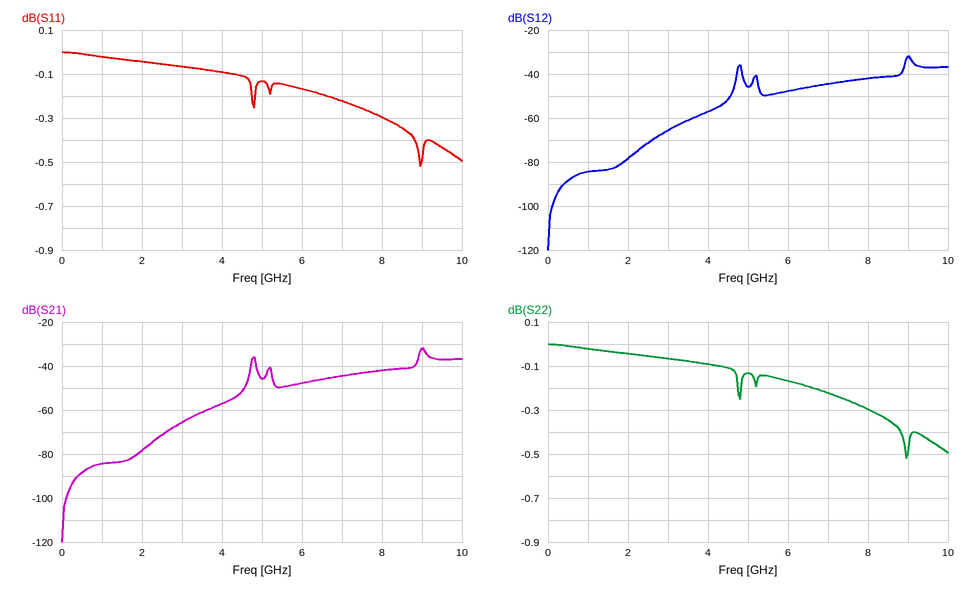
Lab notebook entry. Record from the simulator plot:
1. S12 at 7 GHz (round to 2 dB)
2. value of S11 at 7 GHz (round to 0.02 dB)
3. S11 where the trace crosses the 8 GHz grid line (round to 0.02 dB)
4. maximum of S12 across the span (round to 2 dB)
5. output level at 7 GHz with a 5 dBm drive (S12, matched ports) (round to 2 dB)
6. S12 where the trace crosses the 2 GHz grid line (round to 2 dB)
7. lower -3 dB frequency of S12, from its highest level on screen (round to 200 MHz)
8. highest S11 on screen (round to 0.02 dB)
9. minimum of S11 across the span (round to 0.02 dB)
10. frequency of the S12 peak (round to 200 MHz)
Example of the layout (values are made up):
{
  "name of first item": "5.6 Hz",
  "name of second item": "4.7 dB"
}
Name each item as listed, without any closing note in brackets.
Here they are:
{
  "S12 at 7 GHz": "-44 dB",
  "value of S11 at 7 GHz": "-0.22 dB",
  "S11 where the trace crosses the 8 GHz grid line": "-0.30 dB",
  "maximum of S12 across the span": "-32 dB",
  "output level at 7 GHz with a 5 dBm drive (S12, matched ports)": "-40 dBm",
  "S12 where the trace crosses the 2 GHz grid line": "-78 dB",
  "lower -3 dB frequency of S12, from its highest level on screen": "9.0 GHz",
  "highest S11 on screen": "0.00 dB",
  "minimum of S11 across the span": "-0.52 dB",
  "frequency of the S12 peak": "9.0 GHz"
}
